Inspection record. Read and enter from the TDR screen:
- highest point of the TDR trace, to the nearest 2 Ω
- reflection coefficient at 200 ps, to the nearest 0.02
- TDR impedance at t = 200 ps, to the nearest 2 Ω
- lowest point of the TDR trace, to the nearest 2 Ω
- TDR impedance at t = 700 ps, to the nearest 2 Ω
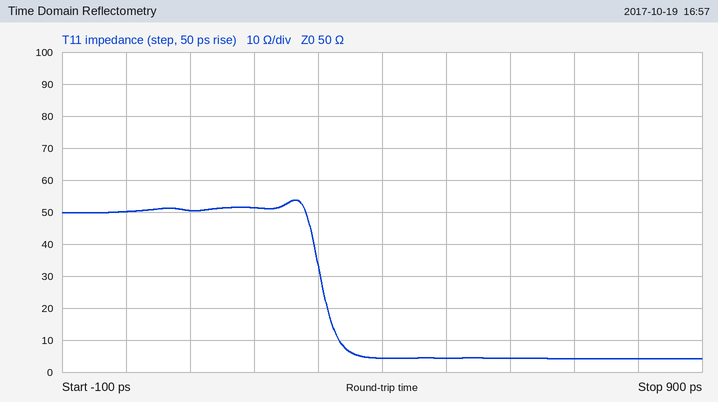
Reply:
54 Ω
+0.02
52 Ω
4 Ω
4 Ω
